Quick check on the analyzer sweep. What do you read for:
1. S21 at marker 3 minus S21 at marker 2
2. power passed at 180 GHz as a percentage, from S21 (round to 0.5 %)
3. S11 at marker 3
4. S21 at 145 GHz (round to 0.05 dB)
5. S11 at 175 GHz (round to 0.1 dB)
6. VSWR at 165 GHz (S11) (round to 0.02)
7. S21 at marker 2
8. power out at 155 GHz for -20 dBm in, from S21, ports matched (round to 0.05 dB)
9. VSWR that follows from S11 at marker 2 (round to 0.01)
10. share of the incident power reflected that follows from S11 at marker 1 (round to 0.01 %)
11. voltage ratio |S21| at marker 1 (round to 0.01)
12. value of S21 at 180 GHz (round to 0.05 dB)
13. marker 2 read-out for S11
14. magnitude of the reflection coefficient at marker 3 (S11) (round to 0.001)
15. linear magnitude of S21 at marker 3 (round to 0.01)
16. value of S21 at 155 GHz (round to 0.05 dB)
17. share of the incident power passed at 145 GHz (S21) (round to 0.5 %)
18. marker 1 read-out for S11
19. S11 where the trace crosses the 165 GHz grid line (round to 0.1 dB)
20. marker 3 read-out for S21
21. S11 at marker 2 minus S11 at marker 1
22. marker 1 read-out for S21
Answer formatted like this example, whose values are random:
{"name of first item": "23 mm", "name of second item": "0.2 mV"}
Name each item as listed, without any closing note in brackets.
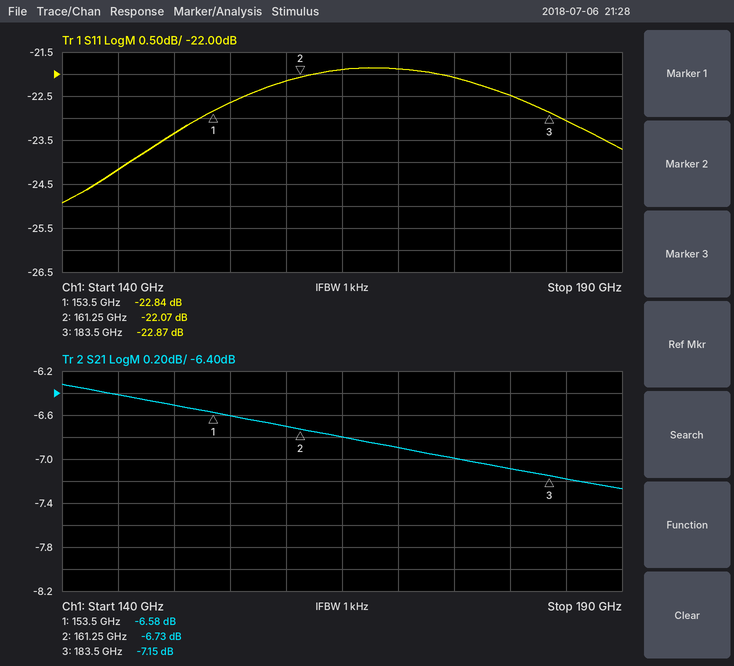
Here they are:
{"S21 at marker 3 minus S21 at marker 2": "-0.42 dB", "power passed at 180 GHz as a percentage, from S21": "19.5 %", "S11 at marker 3": "-22.87 dB", "S21 at 145 GHz": "-6.40 dB", "S11 at 175 GHz": "-22.1 dB", "VSWR at 165 GHz (S11)": "1.18", "S21 at marker 2": "-6.73 dB", "power out at 155 GHz for -20 dBm in, from S21, ports matched": "-26.60 dBm", "VSWR that follows from S11 at marker 2": "1.17", "share of the incident power reflected that follows from S11 at marker 1": "0.52 %", "voltage ratio |S21| at marker 1": "0.47", "value of S21 at 180 GHz": "-7.10 dB", "marker 2 read-out for S11": "-22.07 dB", "magnitude of the reflection coefficient at marker 3 (S11)": "0.072", "linear magnitude of S21 at marker 3": "0.44", "value of S21 at 155 GHz": "-6.60 dB", "share of the incident power passed at 145 GHz (S21)": "23.0 %", "marker 1 read-out for S11": "-22.84 dB", "S11 where the trace crosses the 165 GHz grid line": "-21.9 dB", "marker 3 read-out for S21": "-7.15 dB", "S11 at marker 2 minus S11 at marker 1": "0.77 dB", "marker 1 read-out for S21": "-6.58 dB"}
